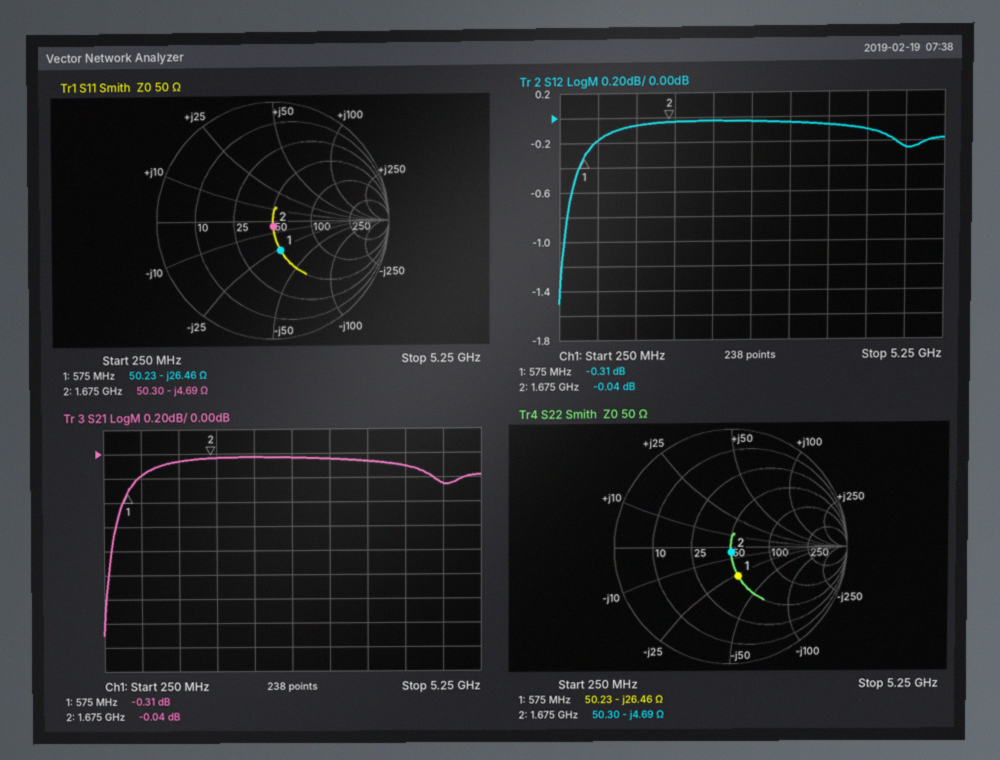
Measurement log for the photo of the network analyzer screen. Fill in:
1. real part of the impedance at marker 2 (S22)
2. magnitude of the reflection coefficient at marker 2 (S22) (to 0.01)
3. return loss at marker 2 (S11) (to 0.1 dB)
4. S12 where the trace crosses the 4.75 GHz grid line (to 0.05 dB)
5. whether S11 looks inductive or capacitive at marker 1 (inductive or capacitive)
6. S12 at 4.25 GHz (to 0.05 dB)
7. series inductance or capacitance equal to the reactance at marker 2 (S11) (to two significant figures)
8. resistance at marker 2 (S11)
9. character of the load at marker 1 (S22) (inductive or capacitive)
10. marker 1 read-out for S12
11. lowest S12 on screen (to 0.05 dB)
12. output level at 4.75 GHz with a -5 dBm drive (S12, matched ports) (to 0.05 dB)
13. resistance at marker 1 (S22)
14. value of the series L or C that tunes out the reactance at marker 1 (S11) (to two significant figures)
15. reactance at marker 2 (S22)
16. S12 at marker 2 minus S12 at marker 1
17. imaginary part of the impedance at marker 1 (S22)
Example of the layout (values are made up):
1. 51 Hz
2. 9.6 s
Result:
1. 50.30 Ω
2. 0.05
3. 26.6 dB
4. -0.25 dB
5. capacitive
6. -0.10 dB
7. 20 pF
8. 50.30 Ω
9. capacitive
10. -0.31 dB
11. -1.50 dB
12. -5.25 dBm
13. 50.23 Ω
14. 7.3 nH
15. -4.69 Ω
16. 0.27 dB
17. -26.46 Ω
